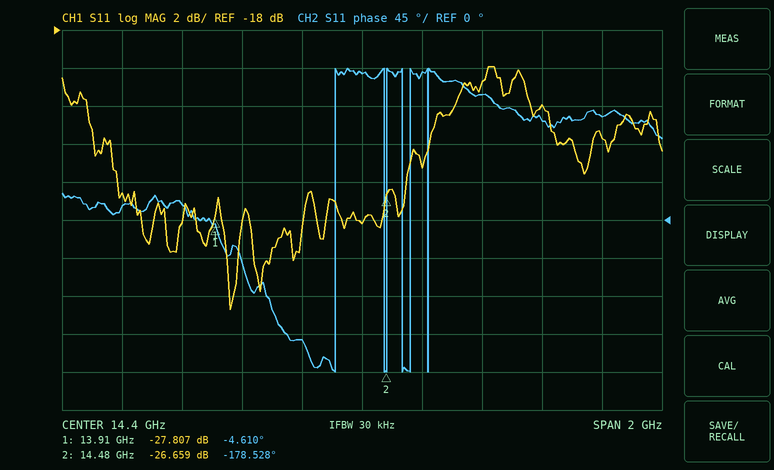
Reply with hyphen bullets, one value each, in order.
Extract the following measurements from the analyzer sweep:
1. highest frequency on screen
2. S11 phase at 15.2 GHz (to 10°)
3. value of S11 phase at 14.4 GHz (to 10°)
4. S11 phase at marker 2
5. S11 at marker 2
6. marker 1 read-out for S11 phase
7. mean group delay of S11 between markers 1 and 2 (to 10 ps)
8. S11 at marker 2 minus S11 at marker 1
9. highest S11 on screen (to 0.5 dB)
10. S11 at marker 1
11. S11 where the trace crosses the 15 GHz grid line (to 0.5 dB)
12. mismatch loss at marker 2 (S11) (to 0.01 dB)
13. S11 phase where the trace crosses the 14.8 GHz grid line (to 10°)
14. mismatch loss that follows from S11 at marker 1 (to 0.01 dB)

- 15.4 GHz
- 120°
- 170°
- -178.528°
- -26.659 dB
- -4.610°
- 850 ps
- 1.148 dB
- -20.0 dB
- -27.807 dB
- -22.0 dB
- 0.01 dB
- 150°
- 0.01 dB
